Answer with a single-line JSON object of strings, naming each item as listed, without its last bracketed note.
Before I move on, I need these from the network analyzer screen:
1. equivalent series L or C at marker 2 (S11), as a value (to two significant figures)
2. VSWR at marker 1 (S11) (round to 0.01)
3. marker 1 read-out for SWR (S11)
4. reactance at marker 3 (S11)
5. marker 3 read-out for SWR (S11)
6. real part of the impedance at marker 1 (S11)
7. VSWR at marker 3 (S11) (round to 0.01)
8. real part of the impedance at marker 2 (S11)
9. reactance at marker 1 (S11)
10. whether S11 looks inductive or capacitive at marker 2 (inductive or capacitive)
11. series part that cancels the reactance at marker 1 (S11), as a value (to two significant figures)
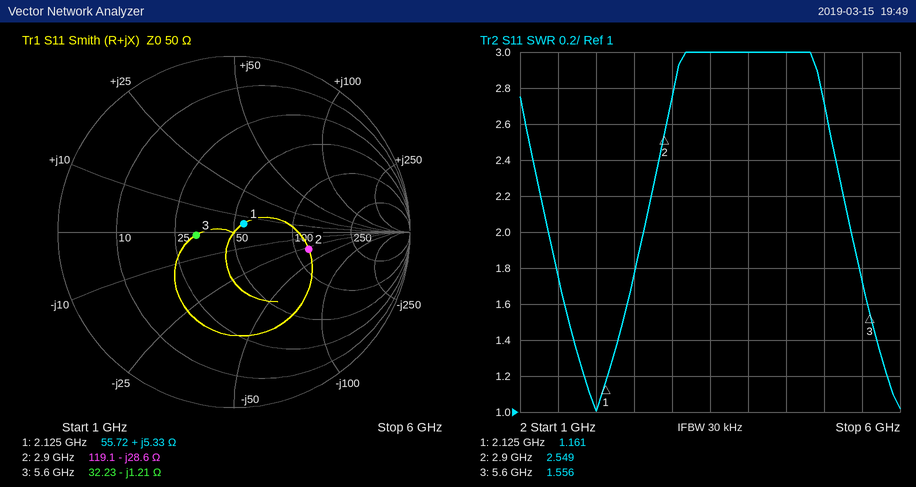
{"equivalent series L or C at marker 2 (S11), as a value": "1.9 pF", "VSWR at marker 1 (S11)": "1.16", "marker 1 read-out for SWR": "1.161", "reactance at marker 3": "-1.21 Ω", "marker 3 read-out for SWR": "1.556", "real part of the impedance at marker 1": "55.72 Ω", "VSWR at marker 3 (S11)": "1.55", "real part of the impedance at marker 2": "119.1 Ω", "reactance at marker 1": "+5.33 Ω", "whether S11 looks inductive or capacitive at marker 2": "capacitive", "series part that cancels the reactance at marker 1 (S11), as a value": "14 pF"}
